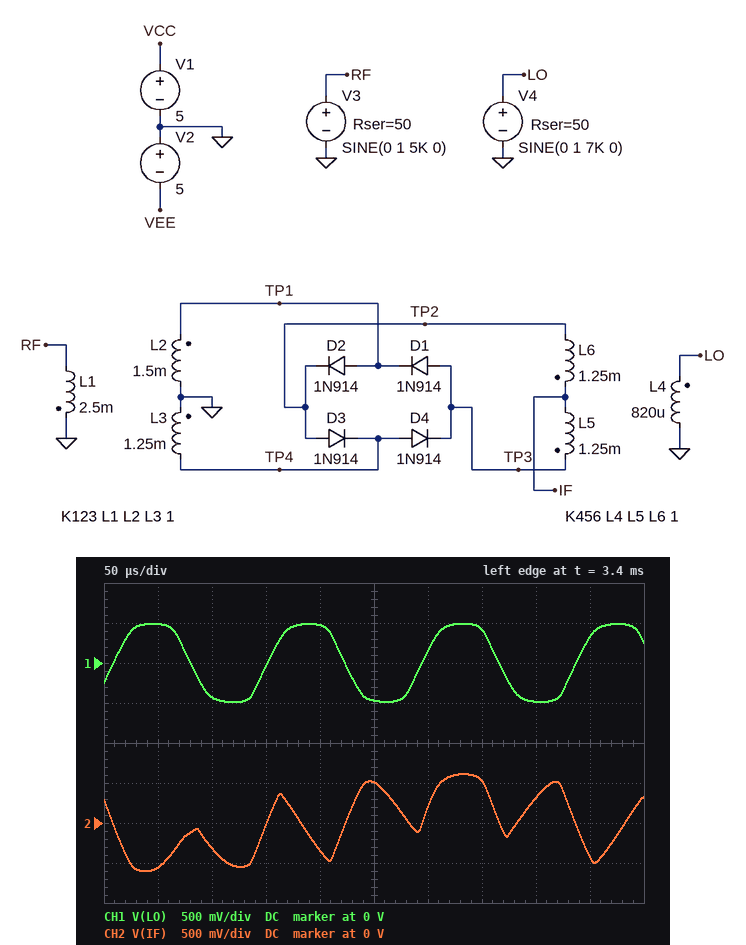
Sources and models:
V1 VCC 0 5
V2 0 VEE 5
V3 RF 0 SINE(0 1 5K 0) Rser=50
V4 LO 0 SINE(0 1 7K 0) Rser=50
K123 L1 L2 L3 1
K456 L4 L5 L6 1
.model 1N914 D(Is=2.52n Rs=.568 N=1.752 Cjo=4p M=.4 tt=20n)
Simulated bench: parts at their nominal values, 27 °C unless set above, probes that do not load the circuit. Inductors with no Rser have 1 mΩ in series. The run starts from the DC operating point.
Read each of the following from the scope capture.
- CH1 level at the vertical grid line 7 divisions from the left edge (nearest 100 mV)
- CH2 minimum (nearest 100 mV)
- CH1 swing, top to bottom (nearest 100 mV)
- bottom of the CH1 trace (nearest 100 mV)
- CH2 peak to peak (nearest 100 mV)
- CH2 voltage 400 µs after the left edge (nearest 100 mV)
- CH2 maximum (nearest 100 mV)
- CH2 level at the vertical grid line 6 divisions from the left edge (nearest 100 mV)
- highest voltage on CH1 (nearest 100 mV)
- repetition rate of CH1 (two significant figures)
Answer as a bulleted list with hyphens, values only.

- 400 mV
- -600 mV
- 1.0 V
- -500 mV
- 1.2 V
- 300 mV
- 600 mV
- 200 mV
- 500 mV
- 7.0 kHz
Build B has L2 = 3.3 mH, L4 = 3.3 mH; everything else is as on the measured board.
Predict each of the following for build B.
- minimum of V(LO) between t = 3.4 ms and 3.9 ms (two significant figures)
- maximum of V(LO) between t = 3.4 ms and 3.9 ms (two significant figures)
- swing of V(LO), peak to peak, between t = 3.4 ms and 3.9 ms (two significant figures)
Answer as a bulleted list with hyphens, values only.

- -930 mV
- 930 mV
- 1.9 V
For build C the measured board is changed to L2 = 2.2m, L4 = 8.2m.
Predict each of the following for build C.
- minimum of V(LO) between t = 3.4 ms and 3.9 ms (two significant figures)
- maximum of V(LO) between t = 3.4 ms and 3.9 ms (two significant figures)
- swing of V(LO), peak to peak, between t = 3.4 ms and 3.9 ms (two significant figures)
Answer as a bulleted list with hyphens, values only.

- -990 mV
- 990 mV
- 2.0 V
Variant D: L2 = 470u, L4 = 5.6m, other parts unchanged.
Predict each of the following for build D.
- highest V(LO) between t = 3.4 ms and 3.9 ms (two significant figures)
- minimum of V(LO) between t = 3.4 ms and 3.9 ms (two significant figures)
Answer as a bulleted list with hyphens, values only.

- 980 mV
- -980 mV
